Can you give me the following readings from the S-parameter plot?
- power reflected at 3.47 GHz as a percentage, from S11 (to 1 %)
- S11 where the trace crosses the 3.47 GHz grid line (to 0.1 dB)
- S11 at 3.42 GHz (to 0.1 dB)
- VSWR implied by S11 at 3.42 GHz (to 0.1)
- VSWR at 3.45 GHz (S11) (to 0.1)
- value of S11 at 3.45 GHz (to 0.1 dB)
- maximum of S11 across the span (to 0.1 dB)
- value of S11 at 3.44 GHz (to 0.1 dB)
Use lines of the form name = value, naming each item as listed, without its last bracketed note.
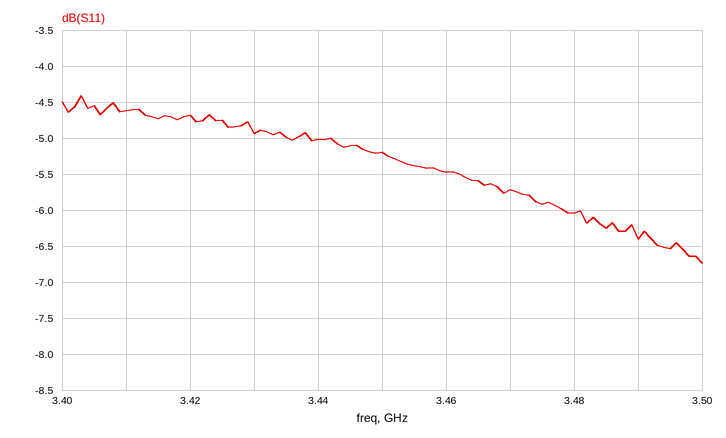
power reflected at 3.47 GHz as a percentage, from S11 = 27 %
S11 where the trace crosses the 3.47 GHz grid line = -5.7 dB
S11 at 3.42 GHz = -4.7 dB
VSWR implied by S11 at 3.42 GHz = 3.8
VSWR at 3.45 GHz (S11) = 3.4
value of S11 at 3.45 GHz = -5.2 dB
maximum of S11 across the span = -4.4 dB
value of S11 at 3.44 GHz = -5.0 dB
